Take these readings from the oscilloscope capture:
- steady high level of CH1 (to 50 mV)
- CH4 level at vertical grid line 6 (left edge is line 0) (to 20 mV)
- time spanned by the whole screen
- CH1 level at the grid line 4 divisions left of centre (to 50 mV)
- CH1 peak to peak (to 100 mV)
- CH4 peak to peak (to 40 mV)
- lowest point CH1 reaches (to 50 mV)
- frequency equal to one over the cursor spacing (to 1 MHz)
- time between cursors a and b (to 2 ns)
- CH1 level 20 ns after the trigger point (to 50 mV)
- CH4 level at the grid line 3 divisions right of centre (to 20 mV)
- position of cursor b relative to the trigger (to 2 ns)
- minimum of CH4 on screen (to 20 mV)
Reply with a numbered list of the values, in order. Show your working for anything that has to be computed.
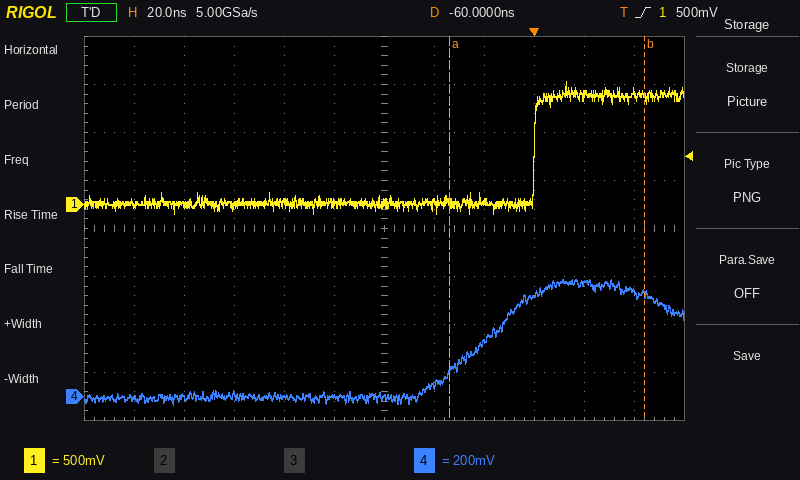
1. 1.15 V
2. 0 mV
3. 240 ns
4. 0 mV
5. 1.40 V
6. 520 mV
7. -100 mV
8. 1 / 78 ns ≈ 13 MHz
9. 78 ns
10. 1.15 V
11. 420 mV
12. +44 ns
13. -40 mV
